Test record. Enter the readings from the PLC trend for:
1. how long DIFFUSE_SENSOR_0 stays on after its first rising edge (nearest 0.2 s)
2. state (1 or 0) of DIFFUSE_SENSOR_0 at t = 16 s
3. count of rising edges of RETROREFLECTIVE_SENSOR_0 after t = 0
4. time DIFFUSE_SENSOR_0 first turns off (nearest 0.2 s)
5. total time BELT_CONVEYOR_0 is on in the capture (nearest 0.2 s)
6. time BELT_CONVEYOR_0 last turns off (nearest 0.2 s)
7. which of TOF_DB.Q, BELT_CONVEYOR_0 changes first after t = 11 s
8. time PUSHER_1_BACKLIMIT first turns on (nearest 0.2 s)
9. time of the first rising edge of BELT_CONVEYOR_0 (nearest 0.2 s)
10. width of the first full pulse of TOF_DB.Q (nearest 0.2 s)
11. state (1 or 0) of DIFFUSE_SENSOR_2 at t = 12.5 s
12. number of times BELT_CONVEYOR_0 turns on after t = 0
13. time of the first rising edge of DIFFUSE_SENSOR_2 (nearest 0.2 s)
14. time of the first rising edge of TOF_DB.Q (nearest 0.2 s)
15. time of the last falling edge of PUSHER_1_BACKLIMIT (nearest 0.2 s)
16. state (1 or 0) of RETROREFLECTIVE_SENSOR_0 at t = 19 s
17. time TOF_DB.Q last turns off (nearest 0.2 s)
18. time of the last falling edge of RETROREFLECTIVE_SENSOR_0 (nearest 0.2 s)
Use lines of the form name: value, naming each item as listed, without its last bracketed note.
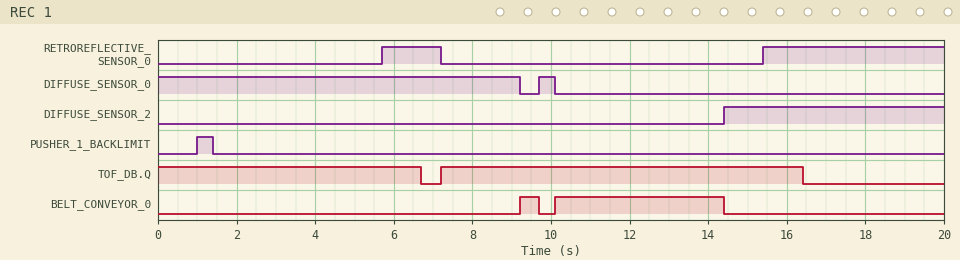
how long DIFFUSE_SENSOR_0 stays on after its first rising edge: 0.4 s
state (1 or 0) of DIFFUSE_SENSOR_0 at t = 16 s: 0
count of rising edges of RETROREFLECTIVE_SENSOR_0 after t = 0: 2
time DIFFUSE_SENSOR_0 first turns off: 9.2 s
total time BELT_CONVEYOR_0 is on in the capture: 4.8 s
time BELT_CONVEYOR_0 last turns off: 14.4 s
which of TOF_DB.Q, BELT_CONVEYOR_0 changes first after t = 11 s: BELT_CONVEYOR_0
time PUSHER_1_BACKLIMIT first turns on: 1.0 s
time of the first rising edge of BELT_CONVEYOR_0: 9.2 s
width of the first full pulse of TOF_DB.Q: 9.2 s
state (1 or 0) of DIFFUSE_SENSOR_2 at t = 12.5 s: 0
number of times BELT_CONVEYOR_0 turns on after t = 0: 2
time of the first rising edge of DIFFUSE_SENSOR_2: 14.4 s
time of the first rising edge of TOF_DB.Q: 7.2 s
time of the last falling edge of PUSHER_1_BACKLIMIT: 1.4 s
state (1 or 0) of RETROREFLECTIVE_SENSOR_0 at t = 19 s: 1
time TOF_DB.Q last turns off: 16.4 s
time of the last falling edge of RETROREFLECTIVE_SENSOR_0: 7.2 s
